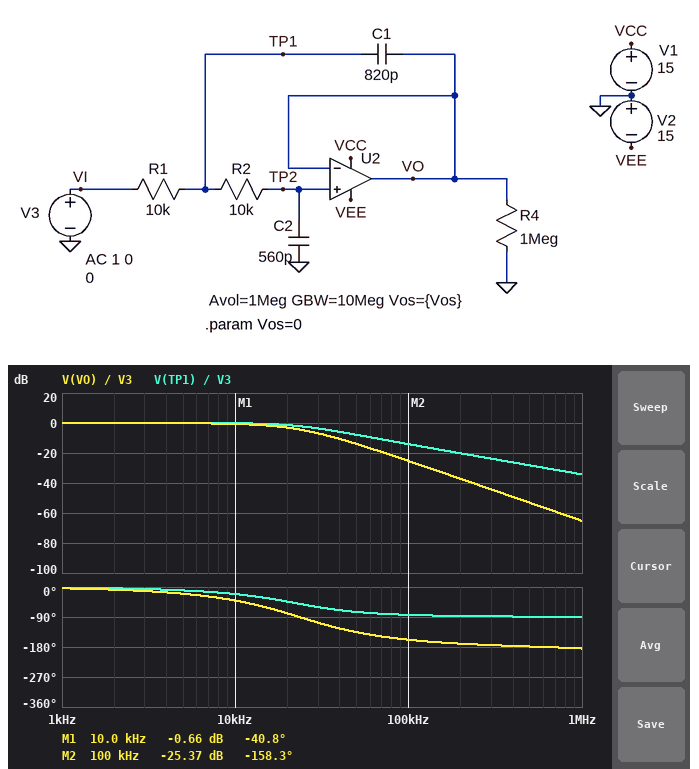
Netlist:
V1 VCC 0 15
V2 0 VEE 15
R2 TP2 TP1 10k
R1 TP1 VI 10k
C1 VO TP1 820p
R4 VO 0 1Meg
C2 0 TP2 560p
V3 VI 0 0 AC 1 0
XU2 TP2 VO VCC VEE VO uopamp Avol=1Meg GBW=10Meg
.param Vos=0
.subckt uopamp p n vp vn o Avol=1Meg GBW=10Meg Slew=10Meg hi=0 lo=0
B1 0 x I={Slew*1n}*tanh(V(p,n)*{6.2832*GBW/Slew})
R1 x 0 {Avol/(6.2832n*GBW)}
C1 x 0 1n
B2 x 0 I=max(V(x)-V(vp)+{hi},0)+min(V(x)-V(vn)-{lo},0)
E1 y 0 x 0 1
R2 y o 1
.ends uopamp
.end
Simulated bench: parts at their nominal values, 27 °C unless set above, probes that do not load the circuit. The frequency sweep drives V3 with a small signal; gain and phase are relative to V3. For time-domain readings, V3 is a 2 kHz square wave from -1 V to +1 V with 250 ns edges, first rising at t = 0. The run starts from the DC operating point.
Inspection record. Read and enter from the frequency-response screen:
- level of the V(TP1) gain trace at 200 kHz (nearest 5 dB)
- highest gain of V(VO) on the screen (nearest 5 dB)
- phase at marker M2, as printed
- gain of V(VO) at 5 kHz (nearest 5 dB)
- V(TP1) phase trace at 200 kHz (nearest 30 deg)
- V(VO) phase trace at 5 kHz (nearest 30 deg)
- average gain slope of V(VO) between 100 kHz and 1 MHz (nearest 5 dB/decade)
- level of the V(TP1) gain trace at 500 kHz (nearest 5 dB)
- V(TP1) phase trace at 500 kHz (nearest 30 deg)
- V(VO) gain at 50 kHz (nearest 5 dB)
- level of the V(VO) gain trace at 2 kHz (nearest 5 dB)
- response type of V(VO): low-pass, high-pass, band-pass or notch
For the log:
-20 dB
0 dB
-158.3 deg
0 dB
-90 deg
-30 deg
-40 dB/decade
-30 dB
-90 deg
-15 dB
0 dB
low-pass
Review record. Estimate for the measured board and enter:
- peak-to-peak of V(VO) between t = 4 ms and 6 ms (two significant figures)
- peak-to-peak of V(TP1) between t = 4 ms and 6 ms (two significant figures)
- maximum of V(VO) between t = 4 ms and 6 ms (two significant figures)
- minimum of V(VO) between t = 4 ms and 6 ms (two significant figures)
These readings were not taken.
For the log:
2.0 V
2.1 V
1.0 V
-1.0 V
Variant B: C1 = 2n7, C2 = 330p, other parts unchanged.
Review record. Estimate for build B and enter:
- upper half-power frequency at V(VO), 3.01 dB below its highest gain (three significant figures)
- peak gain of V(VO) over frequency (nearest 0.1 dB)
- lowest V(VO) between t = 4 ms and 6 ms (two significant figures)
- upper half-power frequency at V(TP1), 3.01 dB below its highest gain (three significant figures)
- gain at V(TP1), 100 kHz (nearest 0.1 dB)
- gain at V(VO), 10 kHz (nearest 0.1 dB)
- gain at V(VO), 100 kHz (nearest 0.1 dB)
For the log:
20.0 kHz
3.7 dB
-1.6 V
20.3 kHz
-23.5 dB
2.3 dB
-30.8 dB
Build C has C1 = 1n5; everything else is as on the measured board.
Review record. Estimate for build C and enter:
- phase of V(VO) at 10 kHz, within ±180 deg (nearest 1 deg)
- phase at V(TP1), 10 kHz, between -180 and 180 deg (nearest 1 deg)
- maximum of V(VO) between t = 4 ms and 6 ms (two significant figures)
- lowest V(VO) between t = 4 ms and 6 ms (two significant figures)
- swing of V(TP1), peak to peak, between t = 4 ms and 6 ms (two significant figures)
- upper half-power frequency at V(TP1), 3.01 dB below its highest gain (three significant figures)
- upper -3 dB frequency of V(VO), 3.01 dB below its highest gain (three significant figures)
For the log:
-47 deg
-27 deg
1.2 V
-1.2 V
2.5 V
21.6 kHz
19.2 kHz
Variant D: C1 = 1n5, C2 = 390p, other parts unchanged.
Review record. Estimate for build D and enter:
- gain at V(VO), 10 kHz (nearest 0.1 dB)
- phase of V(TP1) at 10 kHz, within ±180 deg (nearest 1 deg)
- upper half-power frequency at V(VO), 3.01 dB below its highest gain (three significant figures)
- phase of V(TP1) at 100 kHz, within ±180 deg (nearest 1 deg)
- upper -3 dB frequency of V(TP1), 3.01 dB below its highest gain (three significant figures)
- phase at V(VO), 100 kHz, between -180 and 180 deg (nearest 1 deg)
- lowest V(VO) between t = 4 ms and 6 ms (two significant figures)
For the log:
0.8 dB
-19 deg
24.2 kHz
-100 deg
25.8 kHz
-168 deg
-1.3 V
